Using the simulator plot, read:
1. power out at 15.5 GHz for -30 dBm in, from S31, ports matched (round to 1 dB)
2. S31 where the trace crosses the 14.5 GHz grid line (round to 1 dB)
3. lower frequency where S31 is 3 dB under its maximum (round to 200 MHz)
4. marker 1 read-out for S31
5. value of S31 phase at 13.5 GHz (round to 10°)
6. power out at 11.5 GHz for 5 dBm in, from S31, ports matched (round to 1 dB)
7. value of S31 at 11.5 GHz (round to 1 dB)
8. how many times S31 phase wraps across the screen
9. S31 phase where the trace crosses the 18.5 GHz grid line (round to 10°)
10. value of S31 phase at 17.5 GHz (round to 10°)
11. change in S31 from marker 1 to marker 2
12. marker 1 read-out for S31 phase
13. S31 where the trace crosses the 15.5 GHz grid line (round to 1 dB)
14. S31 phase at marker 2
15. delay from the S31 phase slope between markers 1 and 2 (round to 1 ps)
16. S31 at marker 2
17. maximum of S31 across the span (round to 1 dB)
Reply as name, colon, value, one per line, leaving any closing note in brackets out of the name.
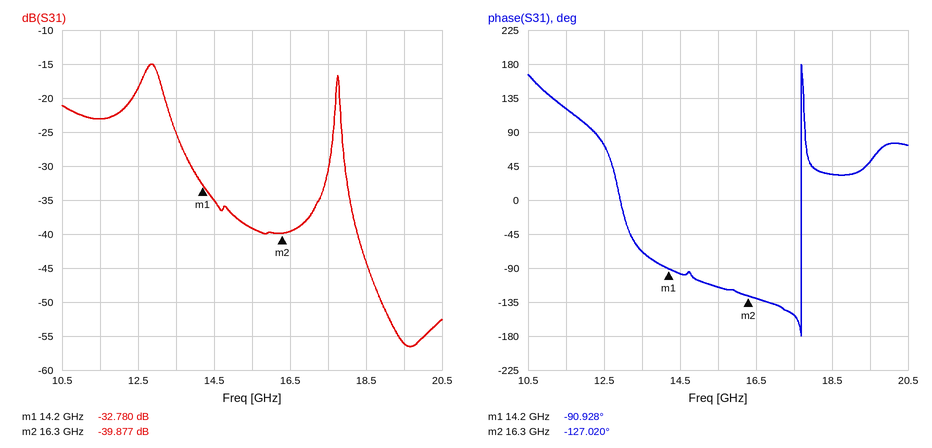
power out at 15.5 GHz for -30 dBm in, from S31, ports matched: -69 dBm
S31 where the trace crosses the 14.5 GHz grid line: -35 dB
lower frequency where S31 is 3 dB under its maximum: 12.6 GHz
marker 1 read-out for S31: -32.780 dB
value of S31 phase at 13.5 GHz: -70°
power out at 11.5 GHz for 5 dBm in, from S31, ports matched: -18 dBm
value of S31 at 11.5 GHz: -23 dB
how many times S31 phase wraps across the screen: 1
S31 phase where the trace crosses the 18.5 GHz grid line: 30°
value of S31 phase at 17.5 GHz: -150°
change in S31 from marker 1 to marker 2: -7.097 dB
marker 1 read-out for S31 phase: -90.928°
S31 where the trace crosses the 15.5 GHz grid line: -39 dB
S31 phase at marker 2: -127.020°
delay from the S31 phase slope between markers 1 and 2: 48 ps
S31 at marker 2: -39.877 dB
maximum of S31 across the span: -15 dB
